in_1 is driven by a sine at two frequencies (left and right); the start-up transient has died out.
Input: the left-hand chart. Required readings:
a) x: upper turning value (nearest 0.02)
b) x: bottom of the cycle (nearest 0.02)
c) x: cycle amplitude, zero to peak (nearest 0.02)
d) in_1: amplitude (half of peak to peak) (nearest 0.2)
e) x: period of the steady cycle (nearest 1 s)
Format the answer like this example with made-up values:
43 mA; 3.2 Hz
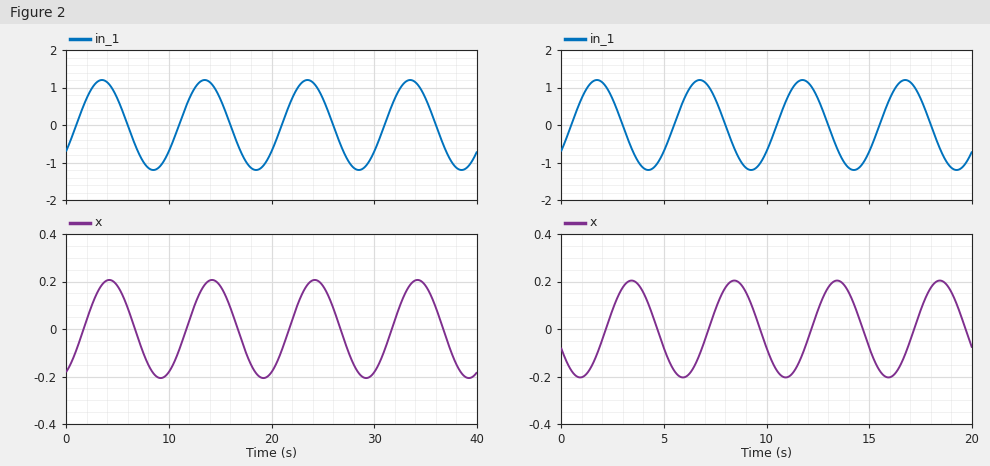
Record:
0.20; -0.20; 0.20; 1.2; 10 s
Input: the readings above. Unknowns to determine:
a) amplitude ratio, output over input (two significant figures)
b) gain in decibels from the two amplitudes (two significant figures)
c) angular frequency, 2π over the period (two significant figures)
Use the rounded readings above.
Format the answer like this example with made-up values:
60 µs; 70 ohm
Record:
0.17; -16 dB; 0.63 rad/s
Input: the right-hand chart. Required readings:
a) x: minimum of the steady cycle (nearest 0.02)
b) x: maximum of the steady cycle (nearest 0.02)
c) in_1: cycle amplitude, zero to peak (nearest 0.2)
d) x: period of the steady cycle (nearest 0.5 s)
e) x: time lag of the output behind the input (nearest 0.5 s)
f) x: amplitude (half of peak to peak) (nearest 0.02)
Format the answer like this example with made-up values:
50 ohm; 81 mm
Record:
-0.20; 0.20; 1.2; 5.0 s; 1.5 s; 0.20
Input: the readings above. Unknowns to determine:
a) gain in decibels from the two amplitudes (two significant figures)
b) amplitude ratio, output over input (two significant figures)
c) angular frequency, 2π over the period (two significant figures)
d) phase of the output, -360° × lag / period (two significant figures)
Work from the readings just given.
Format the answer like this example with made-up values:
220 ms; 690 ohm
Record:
-16 dB; 0.17; 1.3 rad/s; -110°
